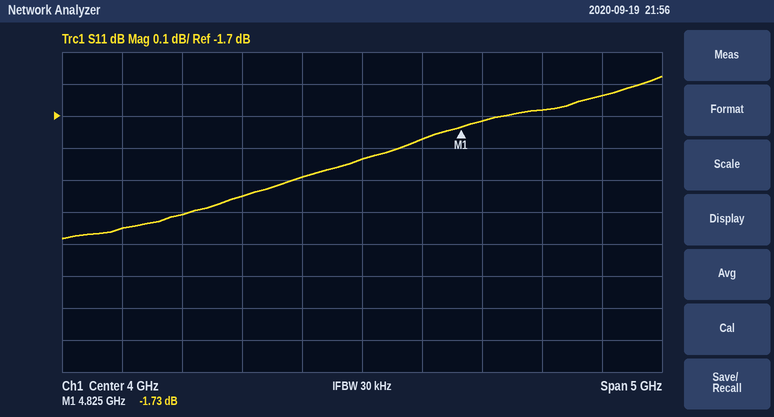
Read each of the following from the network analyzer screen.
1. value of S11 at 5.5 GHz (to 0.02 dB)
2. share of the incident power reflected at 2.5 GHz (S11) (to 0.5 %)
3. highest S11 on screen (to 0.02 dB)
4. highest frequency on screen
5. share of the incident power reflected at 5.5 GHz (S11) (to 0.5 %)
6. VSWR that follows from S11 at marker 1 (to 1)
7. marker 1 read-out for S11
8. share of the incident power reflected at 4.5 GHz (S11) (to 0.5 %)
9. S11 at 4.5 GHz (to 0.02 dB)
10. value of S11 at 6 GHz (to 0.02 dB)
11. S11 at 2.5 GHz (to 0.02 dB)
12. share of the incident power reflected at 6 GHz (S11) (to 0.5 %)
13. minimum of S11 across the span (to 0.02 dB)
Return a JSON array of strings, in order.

["-1.68 dB", "63.0 %", "-1.58 dB", "6.5 GHz", "68.0 %", "10", "-1.73 dB", "66.5 %", "-1.78 dB", "-1.64 dB", "-2.00 dB", "68.5 %", "-2.08 dB"]
